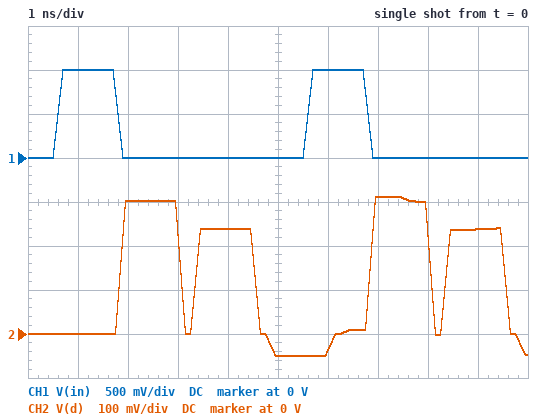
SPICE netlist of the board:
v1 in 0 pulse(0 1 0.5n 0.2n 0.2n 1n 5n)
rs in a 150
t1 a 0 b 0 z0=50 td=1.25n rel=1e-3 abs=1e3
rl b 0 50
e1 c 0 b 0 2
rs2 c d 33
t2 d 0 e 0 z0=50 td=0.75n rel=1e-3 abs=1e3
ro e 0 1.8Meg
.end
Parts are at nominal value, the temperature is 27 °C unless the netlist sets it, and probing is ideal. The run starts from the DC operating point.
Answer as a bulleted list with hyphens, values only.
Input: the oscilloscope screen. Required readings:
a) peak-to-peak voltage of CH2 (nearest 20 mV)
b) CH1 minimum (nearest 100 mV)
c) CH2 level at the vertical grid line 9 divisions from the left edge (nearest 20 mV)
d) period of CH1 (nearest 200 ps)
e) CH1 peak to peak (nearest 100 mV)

- 360 mV
- 0 V
- 240 mV
- 5.0 ns
- 1.0 V
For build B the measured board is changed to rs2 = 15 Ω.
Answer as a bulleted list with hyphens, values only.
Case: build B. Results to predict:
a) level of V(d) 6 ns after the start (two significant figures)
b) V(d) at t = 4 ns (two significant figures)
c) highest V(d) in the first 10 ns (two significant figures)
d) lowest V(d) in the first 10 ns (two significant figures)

- -72 mV
- 180 mV
- 440 mV
- -96 mV
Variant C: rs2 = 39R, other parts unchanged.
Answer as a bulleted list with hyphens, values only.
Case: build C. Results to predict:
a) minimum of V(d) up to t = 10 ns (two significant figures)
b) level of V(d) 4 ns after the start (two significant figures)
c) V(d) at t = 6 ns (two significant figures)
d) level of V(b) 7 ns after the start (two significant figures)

- -30 mV
- 250 mV
- -23 mV
- 250 mV
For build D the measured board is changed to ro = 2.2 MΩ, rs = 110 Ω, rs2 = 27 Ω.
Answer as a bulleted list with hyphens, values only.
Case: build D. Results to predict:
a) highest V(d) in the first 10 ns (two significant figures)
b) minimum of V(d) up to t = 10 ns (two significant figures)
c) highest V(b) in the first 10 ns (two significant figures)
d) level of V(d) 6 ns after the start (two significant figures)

- 430 mV
- -85 mV
- 310 mV
- -64 mV
